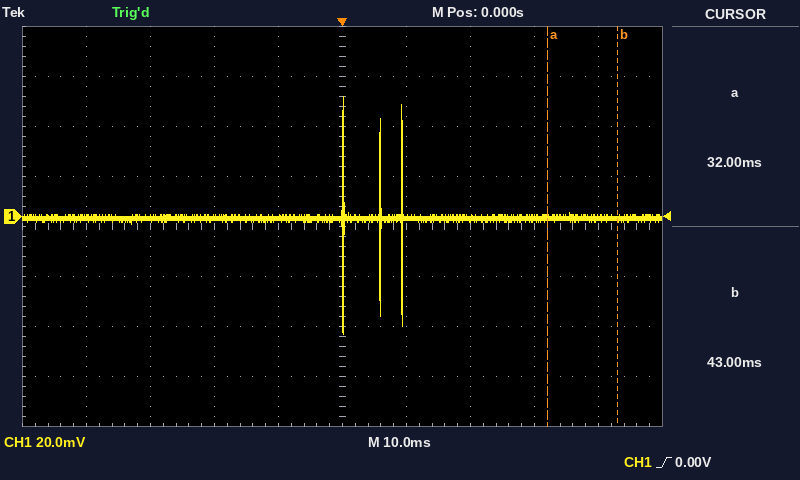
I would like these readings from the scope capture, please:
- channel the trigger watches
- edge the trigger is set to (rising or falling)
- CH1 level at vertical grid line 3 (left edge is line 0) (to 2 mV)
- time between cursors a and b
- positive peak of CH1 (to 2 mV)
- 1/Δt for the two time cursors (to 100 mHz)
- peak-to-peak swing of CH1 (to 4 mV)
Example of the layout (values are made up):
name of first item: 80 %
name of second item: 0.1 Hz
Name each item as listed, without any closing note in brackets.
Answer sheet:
channel the trigger watches: CH1
edge the trigger is set to: rising
CH1 level at vertical grid line 3 (left edge is line 0): 0 mV
time between cursors a and b: 11 ms
positive peak of CH1: 48 mV
1/Δt for the two time cursors: 90.9 Hz
peak-to-peak swing of CH1: 96 mV
